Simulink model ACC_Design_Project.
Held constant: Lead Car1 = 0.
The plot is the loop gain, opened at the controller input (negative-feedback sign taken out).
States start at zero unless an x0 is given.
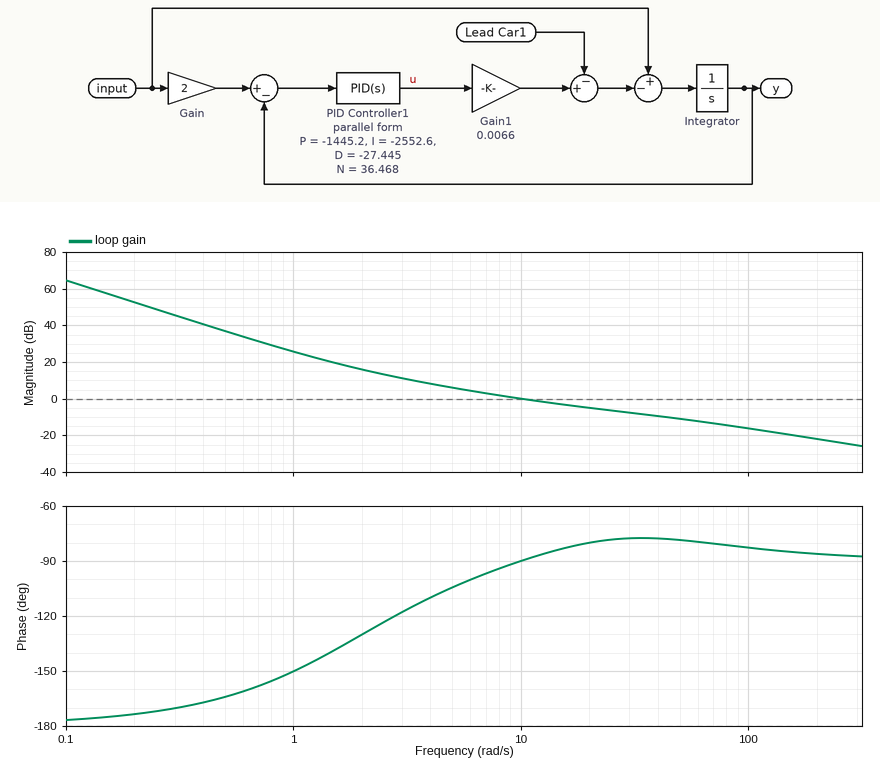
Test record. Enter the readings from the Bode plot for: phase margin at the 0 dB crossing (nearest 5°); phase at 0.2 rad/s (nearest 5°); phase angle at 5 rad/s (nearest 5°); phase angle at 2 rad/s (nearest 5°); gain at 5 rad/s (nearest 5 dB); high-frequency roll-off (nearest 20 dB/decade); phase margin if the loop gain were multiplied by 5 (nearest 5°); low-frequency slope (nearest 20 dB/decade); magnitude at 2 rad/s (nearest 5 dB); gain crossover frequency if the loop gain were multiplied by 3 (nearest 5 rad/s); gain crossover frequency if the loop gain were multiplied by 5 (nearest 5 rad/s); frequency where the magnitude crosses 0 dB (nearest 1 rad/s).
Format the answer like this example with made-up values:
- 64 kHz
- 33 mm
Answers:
- 90°
- -175°
- -105°
- -130°
- 5 dB
- -20 dB/decade
- 100°
- -40 dB/decade
- 15 dB
- 40 rad/s
- 75 rad/s
- 10 rad/s
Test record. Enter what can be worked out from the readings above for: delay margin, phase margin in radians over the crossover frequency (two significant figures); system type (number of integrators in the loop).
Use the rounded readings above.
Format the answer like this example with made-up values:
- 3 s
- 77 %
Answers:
- 0.16 s
- 2
